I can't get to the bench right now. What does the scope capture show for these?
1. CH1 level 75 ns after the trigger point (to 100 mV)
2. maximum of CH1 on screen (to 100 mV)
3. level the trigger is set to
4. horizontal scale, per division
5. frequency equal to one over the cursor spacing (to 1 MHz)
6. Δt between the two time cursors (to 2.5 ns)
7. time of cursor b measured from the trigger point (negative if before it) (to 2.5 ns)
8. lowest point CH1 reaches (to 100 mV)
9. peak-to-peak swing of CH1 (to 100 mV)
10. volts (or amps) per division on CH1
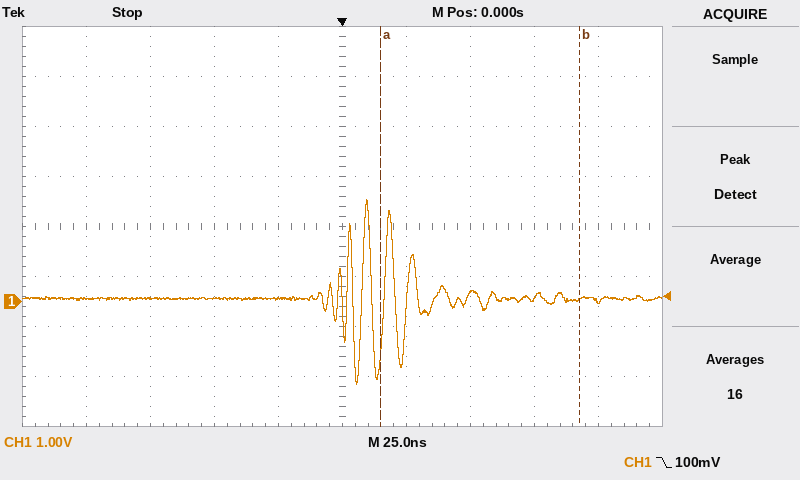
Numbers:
100 mV
2.0 V
100 mV
25 ns
13 MHz
77.5 ns
+92.5 ns
-1.7 V
3.7 V
1 V
